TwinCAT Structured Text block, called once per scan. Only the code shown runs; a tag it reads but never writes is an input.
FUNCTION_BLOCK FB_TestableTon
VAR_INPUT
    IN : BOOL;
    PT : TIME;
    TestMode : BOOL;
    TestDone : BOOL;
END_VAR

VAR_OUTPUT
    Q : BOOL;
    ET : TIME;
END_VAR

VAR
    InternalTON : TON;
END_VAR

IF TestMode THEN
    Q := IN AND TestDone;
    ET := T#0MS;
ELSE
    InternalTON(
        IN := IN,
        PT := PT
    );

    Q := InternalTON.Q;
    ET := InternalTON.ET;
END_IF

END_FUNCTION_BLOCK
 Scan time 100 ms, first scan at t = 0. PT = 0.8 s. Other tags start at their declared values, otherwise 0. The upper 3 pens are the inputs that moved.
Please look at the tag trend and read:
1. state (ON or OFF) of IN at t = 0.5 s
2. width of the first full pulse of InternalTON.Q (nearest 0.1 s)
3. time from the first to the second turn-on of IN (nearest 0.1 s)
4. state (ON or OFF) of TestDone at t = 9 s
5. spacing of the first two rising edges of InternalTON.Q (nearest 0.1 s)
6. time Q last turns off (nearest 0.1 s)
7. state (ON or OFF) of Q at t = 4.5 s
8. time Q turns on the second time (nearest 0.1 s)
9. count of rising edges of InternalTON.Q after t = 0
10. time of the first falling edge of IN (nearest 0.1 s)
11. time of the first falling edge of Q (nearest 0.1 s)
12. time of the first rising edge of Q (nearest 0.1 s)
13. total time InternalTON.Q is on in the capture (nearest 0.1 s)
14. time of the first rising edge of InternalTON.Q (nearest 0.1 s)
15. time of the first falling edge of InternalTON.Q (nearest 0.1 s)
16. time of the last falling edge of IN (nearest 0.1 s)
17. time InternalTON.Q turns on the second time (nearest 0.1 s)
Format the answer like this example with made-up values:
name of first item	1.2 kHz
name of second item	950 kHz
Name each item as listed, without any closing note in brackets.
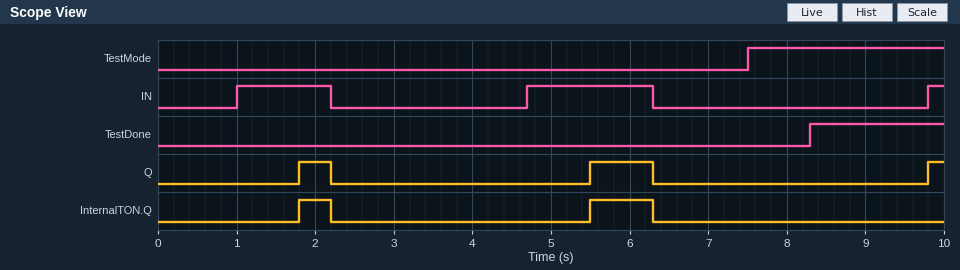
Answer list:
state (ON or OFF) of IN at t = 0.5 s	OFF
width of the first full pulse of InternalTON.Q	0.4 s
time from the first to the second turn-on of IN	3.7 s
state (ON or OFF) of TestDone at t = 9 s	ON
spacing of the first two rising edges of InternalTON.Q	3.7 s
time Q last turns off	6.3 s
state (ON or OFF) of Q at t = 4.5 s	OFF
time Q turns on the second time	5.5 s
count of rising edges of InternalTON.Q after t = 0	2
time of the first falling edge of IN	2.2 s
time of the first falling edge of Q	2.2 s
time of the first rising edge of Q	1.8 s
total time InternalTON.Q is on in the capture	1.2 s
time of the first rising edge of InternalTON.Q	1.8 s
time of the first falling edge of InternalTON.Q	2.2 s
time of the last falling edge of IN	6.3 s
time InternalTON.Q turns on the second time	5.5 s
